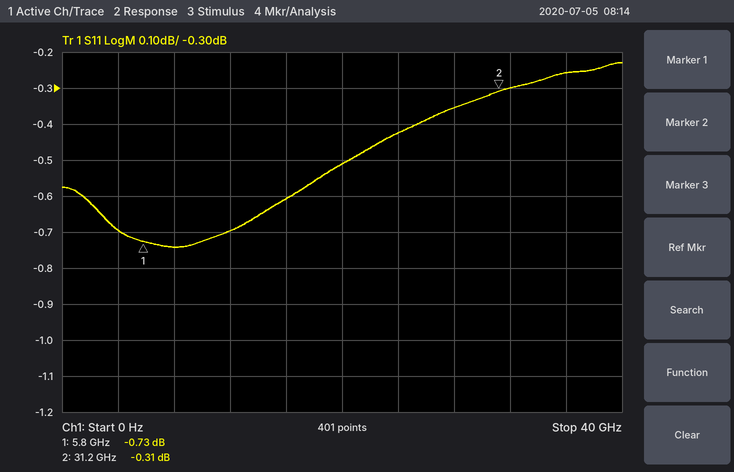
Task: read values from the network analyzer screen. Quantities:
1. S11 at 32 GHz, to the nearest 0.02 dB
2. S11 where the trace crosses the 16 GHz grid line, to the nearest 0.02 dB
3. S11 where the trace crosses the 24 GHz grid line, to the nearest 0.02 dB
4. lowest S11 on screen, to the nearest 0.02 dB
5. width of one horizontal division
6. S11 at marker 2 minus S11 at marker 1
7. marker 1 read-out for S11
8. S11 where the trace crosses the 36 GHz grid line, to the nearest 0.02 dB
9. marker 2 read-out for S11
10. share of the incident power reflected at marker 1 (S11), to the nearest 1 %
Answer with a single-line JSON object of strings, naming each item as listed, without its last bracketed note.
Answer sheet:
{"S11 at 32 GHz, to the nearest 0.02 dB": "-0.30 dB", "S11 where the trace crosses the 16 GHz grid line, to the nearest 0.02 dB": "-0.60 dB", "S11 where the trace crosses the 24 GHz grid line, to the nearest 0.02 dB": "-0.42 dB", "lowest S11 on screen, to the nearest 0.02 dB": "-0.74 dB", "width of one horizontal division": "4 GHz", "S11 at marker 2 minus S11 at marker 1": "0.42 dB", "marker 1 read-out for S11": "-0.73 dB", "S11 where the trace crosses the 36 GHz grid line, to the nearest 0.02 dB": "-0.26 dB", "marker 2 read-out for S11": "-0.31 dB", "share of the incident power reflected at marker 1 (S11), to the nearest 1 %": "85 %"}
